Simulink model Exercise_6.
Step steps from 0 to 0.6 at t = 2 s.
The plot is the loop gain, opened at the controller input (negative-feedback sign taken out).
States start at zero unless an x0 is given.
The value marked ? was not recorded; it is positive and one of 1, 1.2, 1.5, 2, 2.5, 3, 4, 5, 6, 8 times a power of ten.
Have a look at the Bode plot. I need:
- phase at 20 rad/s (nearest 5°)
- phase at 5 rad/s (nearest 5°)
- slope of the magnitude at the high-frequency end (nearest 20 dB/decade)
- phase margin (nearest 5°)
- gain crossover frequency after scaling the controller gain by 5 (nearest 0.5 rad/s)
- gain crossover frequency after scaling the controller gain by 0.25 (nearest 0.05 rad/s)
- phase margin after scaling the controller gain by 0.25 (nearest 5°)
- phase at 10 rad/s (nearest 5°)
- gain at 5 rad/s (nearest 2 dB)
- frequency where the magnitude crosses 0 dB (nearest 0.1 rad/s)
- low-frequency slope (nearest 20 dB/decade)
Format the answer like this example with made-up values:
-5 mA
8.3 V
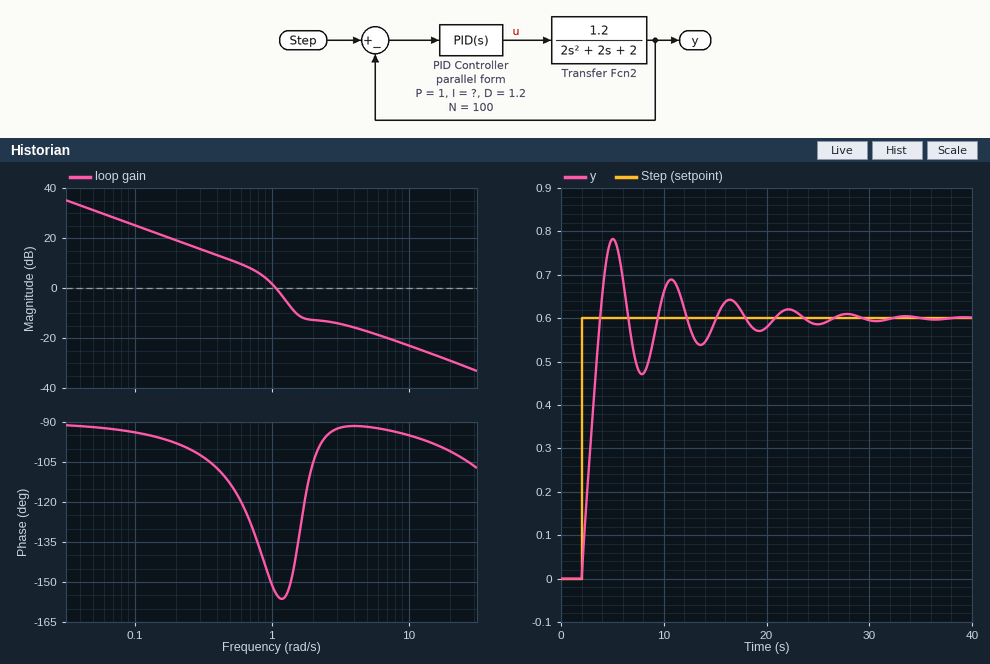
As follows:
-100°
-90°
-20 dB/decade
25°
3.0 rad/s
0.45 rad/s
70°
-95°
-18 dB
1.1 rad/s
-20 dB/decade
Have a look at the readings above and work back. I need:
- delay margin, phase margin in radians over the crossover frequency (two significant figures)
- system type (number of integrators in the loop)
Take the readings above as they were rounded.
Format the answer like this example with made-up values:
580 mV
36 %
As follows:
0.40 s
1
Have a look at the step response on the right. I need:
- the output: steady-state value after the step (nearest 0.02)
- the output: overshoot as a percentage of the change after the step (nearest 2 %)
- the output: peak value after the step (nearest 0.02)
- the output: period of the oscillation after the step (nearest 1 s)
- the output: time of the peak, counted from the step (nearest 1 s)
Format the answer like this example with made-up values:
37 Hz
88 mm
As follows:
0.60
30 %
0.78
6 s
3 s
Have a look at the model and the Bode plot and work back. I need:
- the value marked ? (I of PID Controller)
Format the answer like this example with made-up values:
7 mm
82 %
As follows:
3
